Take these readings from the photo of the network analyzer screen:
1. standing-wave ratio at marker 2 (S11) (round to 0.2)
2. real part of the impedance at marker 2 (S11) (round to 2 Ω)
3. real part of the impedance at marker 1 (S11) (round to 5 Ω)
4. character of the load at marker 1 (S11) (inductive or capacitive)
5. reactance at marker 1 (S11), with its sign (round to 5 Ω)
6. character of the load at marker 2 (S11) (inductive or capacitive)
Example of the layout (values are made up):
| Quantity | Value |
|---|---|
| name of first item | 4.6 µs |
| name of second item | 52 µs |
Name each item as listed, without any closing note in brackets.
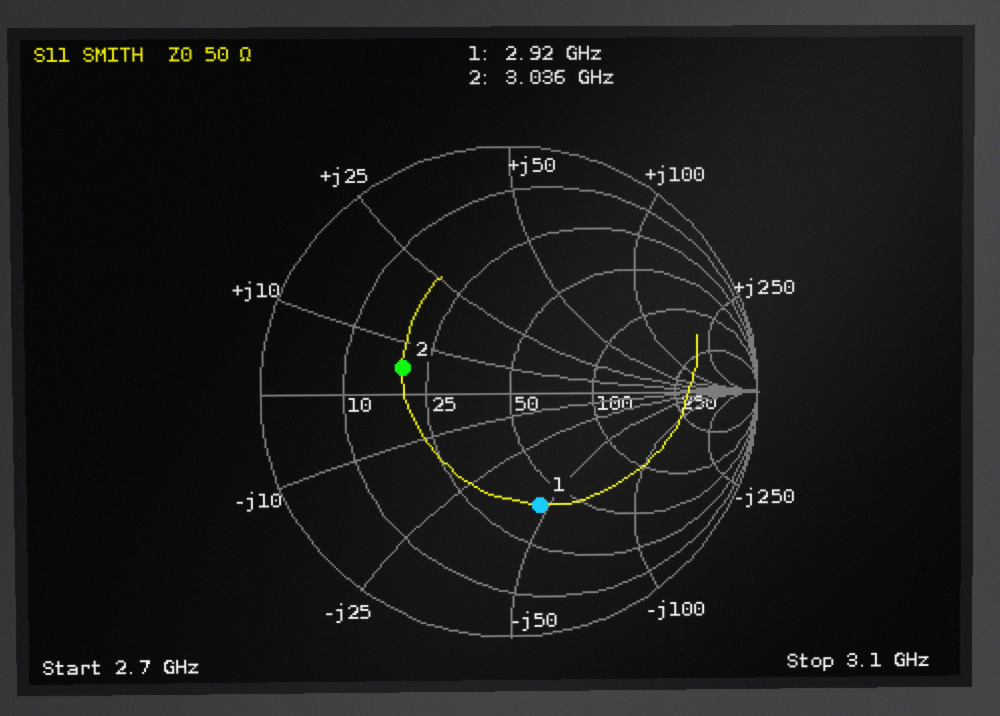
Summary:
| Quantity | Value |
|---|---|
| standing-wave ratio at marker 2 (S11) | 2.6 |
| real part of the impedance at marker 2 (S11) | 20 Ω |
| real part of the impedance at marker 1 (S11) | 40 Ω |
| character of the load at marker 1 (S11) | capacitive |
| reactance at marker 1 (S11), with its sign | -45 Ω |
| character of the load at marker 2 (S11) | inductive |
